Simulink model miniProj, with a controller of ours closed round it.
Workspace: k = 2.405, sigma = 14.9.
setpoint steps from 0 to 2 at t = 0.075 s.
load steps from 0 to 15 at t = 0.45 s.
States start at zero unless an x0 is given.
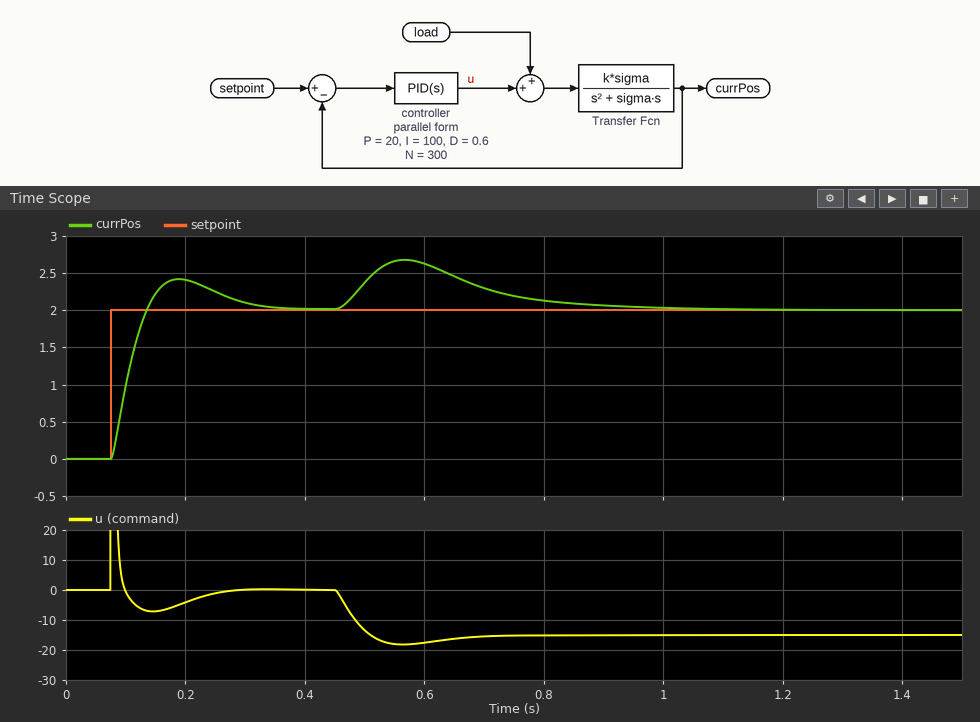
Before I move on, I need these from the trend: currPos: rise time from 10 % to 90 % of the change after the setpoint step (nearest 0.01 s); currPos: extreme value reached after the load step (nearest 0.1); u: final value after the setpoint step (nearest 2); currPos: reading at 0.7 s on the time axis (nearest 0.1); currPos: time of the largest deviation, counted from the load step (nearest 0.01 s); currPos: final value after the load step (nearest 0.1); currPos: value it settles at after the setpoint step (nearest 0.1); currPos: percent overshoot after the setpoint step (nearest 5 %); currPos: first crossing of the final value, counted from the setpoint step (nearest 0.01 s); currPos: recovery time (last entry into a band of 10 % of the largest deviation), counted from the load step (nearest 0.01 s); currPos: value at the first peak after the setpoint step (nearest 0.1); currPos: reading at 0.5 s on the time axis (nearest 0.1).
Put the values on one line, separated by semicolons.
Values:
0.04 s; 2.7; 0; 2.3; 0.12 s; 2.0; 2.0; 20 %; 0.06 s; 0.45 s; 2.4; 2.4
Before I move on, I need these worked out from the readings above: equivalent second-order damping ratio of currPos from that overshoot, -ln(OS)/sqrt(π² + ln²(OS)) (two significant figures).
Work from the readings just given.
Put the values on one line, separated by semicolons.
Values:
0.46
